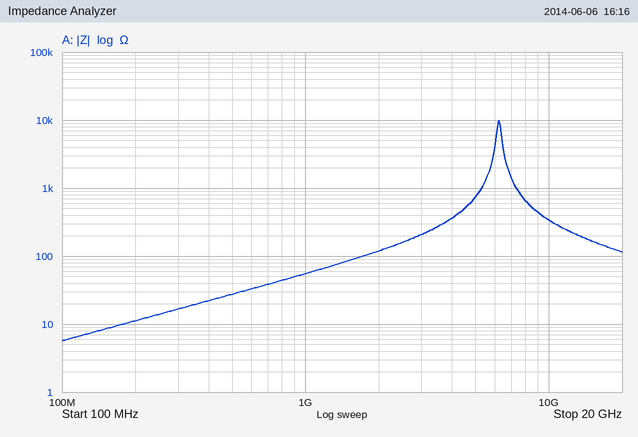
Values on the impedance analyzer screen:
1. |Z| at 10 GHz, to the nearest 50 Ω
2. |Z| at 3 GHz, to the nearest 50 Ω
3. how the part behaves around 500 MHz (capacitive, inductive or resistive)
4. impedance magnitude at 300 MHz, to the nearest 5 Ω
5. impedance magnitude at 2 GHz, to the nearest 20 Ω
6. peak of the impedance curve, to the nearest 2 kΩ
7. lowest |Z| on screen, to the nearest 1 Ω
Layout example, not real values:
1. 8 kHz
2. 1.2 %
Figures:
1. 350 Ω
2. 200 Ω
3. inductive
4. 15 Ω
5. 120 Ω
6. 10 kΩ
7. 6 Ω
